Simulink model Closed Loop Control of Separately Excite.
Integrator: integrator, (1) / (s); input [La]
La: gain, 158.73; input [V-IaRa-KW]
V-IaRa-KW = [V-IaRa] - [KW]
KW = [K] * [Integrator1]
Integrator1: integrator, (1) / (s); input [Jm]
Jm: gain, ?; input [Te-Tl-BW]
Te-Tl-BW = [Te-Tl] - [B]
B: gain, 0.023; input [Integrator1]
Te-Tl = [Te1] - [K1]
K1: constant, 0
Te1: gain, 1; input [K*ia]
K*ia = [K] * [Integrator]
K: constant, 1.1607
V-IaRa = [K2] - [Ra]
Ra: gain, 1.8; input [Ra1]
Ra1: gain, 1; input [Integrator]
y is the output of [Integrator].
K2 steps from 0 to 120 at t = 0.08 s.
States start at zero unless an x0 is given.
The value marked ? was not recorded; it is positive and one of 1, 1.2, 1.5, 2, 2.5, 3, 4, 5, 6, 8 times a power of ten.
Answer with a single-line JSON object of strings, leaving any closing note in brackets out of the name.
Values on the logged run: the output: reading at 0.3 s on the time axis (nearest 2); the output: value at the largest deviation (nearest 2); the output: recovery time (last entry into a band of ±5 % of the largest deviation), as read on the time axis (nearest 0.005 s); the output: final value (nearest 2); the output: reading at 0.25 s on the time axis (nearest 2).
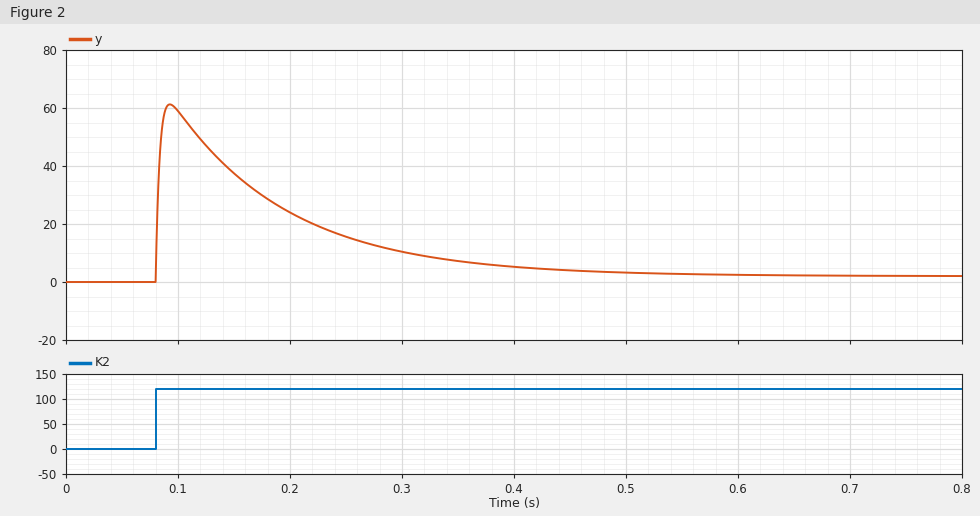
{"the output: reading at 0.3 s on the time axis": "10", "the output: value at the largest deviation": "62", "the output: recovery time (last entry into a band of ±5 % of the largest deviation), as read on the time axis": "0.405 s", "the output: final value": "2", "the output: reading at 0.25 s on the time axis": "16"}
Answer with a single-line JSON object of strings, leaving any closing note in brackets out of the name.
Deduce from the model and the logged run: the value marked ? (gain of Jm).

{"the value marked ?": "12"}
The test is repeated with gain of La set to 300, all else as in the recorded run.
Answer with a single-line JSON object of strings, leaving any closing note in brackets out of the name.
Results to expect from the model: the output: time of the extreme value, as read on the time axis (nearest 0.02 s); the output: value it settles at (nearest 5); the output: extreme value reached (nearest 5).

{"the output: time of the extreme value, as read on the time axis": "0.08 s", "the output: value it settles at": "0", "the output: extreme value reached": "65"}
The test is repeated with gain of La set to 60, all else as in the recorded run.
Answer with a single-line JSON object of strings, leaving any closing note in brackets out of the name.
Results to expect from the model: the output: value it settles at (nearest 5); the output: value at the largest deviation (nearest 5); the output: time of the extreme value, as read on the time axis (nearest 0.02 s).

{"the output: value it settles at": "0", "the output: value at the largest deviation": "55", "the output: time of the extreme value, as read on the time axis": "0.10 s"}
